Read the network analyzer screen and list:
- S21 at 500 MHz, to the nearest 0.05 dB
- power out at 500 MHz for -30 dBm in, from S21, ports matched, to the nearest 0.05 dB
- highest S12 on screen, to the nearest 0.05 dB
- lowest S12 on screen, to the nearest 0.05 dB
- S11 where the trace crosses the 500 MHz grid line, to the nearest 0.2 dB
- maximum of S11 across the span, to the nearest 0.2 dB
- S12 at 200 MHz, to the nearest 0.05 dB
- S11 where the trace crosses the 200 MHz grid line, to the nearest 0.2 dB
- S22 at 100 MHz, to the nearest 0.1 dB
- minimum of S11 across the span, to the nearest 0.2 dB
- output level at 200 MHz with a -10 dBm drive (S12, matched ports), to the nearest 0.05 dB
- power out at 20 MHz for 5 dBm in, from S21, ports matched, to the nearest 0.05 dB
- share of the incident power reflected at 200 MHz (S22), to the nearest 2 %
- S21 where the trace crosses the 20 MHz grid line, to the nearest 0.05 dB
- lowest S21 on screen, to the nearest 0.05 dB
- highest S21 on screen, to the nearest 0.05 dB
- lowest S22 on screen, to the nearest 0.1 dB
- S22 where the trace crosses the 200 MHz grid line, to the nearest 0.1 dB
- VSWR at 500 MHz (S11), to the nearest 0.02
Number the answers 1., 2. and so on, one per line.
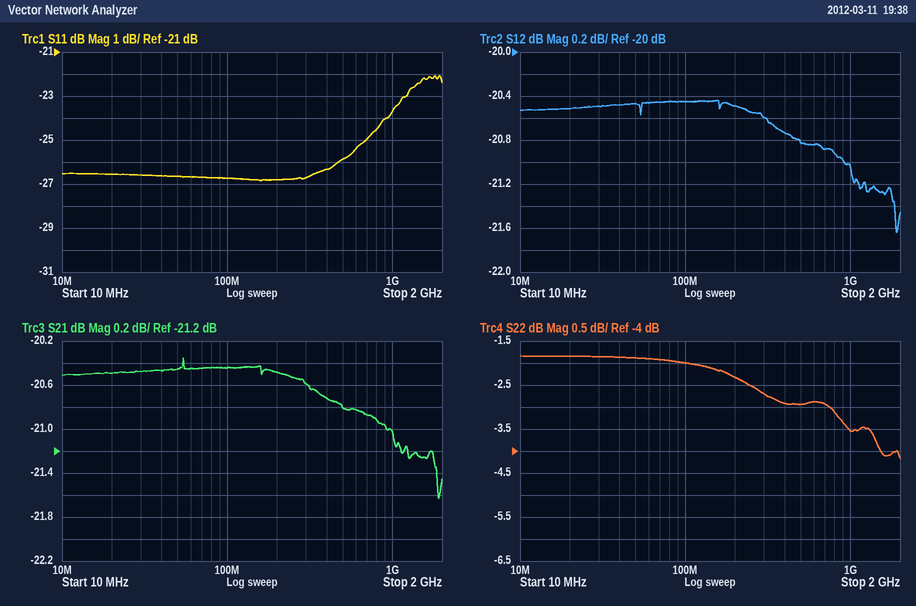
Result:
1. -20.80 dB
2. -50.80 dBm
3. -20.45 dB
4. -21.65 dB
5. -25.8 dB
6. -22.0 dB
7. -20.50 dB
8. -26.8 dB
9. -2.0 dB
10. -26.8 dB
11. -30.50 dBm
12. -15.50 dBm
13. 58 %
14. -20.50 dB
15. -21.65 dB
16. -20.35 dB
17. -4.2 dB
18. -2.3 dB
19. 1.10
